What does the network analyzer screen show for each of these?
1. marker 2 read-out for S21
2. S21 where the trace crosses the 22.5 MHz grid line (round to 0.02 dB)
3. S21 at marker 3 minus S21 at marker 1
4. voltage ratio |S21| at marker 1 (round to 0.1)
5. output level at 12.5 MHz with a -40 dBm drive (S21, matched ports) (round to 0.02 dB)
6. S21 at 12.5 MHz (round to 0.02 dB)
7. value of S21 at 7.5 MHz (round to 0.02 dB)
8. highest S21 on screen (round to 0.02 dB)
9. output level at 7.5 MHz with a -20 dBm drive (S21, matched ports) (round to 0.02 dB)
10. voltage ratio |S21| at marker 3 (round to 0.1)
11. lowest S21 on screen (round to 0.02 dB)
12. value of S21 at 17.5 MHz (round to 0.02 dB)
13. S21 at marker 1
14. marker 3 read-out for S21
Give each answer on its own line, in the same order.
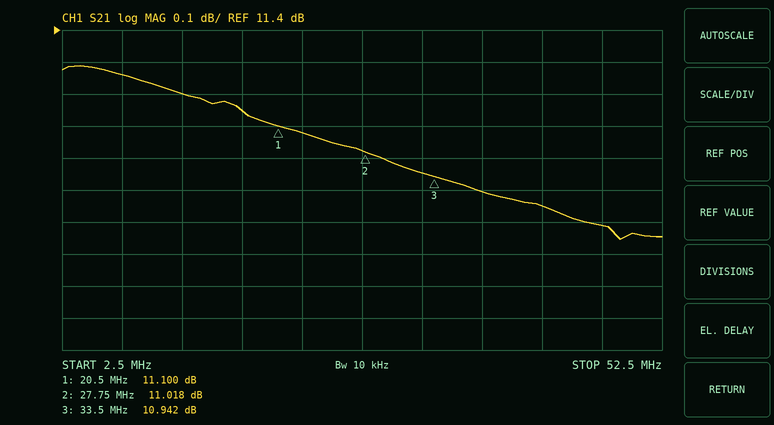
11.018 dB
11.08 dB
-0.158 dB
3.6
-28.80 dBm
11.20 dB
11.26 dB
11.28 dB
-8.74 dBm
3.5
10.74 dB
11.14 dB
11.100 dB
10.942 dB
